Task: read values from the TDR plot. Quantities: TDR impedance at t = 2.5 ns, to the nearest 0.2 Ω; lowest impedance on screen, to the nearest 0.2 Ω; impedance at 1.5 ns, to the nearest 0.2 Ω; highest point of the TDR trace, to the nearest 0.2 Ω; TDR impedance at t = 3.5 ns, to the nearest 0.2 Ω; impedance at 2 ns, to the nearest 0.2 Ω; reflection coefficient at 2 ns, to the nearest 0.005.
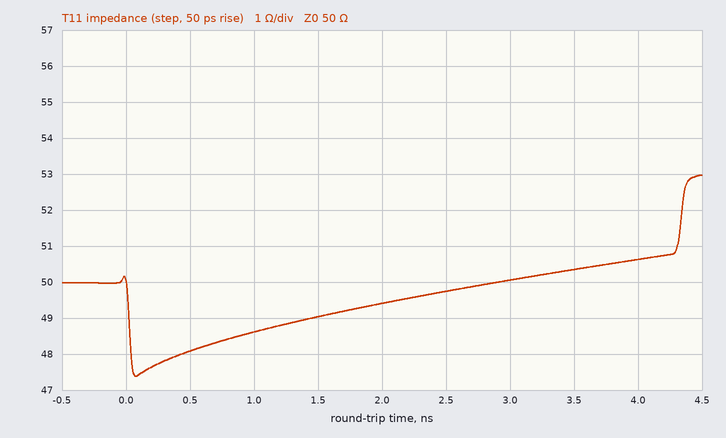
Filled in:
49.8 Ω
47.4 Ω
49.0 Ω
53.0 Ω
50.4 Ω
49.4 Ω
-0.005
